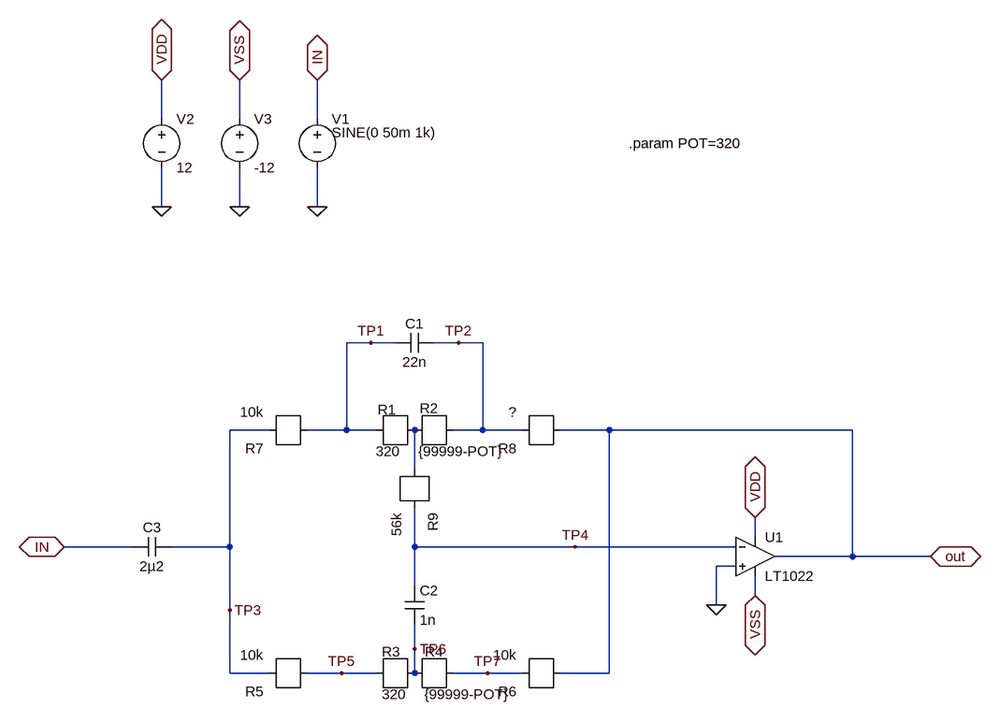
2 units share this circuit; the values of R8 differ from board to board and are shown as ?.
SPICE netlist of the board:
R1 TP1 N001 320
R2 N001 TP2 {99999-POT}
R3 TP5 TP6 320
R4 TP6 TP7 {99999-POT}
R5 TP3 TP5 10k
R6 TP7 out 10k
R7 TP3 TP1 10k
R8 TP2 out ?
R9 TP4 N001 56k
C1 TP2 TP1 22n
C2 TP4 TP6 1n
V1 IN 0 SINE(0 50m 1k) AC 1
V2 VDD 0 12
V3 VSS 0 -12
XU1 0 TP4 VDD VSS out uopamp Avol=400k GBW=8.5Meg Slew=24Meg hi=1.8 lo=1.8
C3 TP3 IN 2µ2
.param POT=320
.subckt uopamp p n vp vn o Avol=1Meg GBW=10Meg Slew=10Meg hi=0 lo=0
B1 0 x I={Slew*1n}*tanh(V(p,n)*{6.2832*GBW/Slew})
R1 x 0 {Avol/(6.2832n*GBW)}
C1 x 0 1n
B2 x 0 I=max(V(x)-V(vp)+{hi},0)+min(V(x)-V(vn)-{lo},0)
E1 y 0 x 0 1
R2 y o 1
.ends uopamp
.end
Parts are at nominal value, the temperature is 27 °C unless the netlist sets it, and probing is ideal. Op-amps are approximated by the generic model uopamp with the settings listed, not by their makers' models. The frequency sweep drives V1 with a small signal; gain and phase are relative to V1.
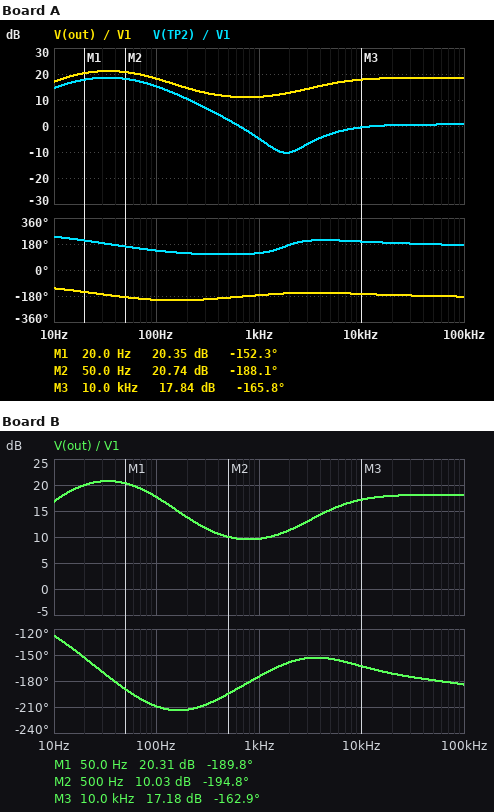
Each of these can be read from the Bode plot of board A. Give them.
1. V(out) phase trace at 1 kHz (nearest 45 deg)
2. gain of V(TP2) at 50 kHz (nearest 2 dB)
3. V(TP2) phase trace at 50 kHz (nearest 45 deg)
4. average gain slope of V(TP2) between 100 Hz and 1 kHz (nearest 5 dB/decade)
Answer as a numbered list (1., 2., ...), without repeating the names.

1. -180 deg
2. 0 dB
3. 180 deg
4. -20 dB/decade
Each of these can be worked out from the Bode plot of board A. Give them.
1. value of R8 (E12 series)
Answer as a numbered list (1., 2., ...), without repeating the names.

1. 33 kΩ
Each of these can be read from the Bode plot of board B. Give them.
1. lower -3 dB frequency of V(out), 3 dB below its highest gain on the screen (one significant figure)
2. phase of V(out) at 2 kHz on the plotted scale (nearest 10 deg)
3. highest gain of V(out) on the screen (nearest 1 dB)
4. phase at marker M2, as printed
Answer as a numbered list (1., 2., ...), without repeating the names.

1. 10 Hz
2. -160 deg
3. 21 dB
4. -194.8 deg
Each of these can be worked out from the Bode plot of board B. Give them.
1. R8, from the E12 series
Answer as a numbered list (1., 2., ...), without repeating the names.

1. 27 kΩ
